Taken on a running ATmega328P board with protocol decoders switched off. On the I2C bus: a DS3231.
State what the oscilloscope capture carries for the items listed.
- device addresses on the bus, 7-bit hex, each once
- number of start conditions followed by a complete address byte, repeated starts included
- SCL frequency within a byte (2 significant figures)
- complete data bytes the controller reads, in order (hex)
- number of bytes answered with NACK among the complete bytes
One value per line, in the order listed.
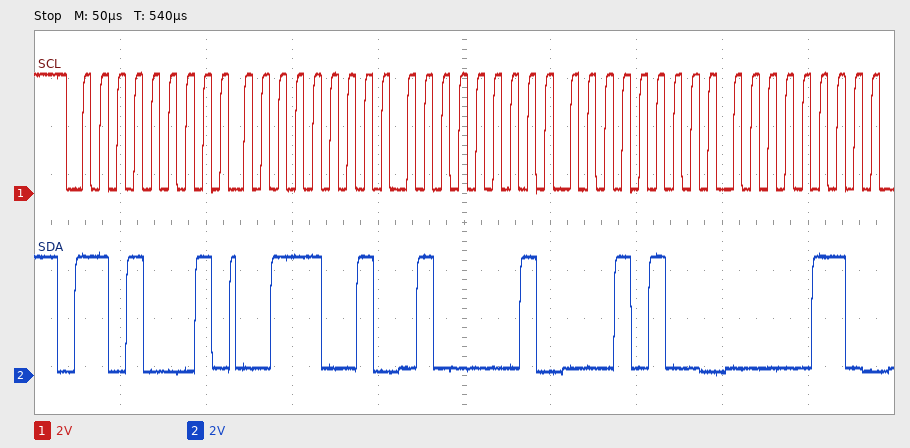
0x68
1
100 kHz
39 41 14 06
0
